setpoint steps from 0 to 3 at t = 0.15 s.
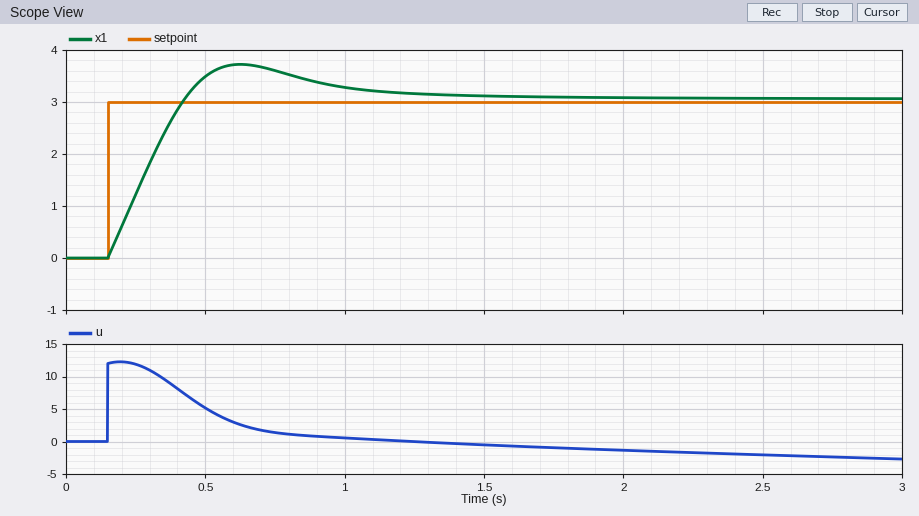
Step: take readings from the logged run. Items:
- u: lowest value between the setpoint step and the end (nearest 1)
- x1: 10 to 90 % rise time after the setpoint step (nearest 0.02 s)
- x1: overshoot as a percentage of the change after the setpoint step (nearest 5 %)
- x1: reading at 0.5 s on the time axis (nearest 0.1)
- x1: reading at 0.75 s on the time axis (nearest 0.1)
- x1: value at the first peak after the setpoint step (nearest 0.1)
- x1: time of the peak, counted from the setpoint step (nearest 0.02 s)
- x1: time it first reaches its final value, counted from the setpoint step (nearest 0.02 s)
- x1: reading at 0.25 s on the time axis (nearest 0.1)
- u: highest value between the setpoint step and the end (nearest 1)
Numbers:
-3
0.22 s
20 %
3.5
3.6
3.7
0.48 s
0.28 s
1.2
12
